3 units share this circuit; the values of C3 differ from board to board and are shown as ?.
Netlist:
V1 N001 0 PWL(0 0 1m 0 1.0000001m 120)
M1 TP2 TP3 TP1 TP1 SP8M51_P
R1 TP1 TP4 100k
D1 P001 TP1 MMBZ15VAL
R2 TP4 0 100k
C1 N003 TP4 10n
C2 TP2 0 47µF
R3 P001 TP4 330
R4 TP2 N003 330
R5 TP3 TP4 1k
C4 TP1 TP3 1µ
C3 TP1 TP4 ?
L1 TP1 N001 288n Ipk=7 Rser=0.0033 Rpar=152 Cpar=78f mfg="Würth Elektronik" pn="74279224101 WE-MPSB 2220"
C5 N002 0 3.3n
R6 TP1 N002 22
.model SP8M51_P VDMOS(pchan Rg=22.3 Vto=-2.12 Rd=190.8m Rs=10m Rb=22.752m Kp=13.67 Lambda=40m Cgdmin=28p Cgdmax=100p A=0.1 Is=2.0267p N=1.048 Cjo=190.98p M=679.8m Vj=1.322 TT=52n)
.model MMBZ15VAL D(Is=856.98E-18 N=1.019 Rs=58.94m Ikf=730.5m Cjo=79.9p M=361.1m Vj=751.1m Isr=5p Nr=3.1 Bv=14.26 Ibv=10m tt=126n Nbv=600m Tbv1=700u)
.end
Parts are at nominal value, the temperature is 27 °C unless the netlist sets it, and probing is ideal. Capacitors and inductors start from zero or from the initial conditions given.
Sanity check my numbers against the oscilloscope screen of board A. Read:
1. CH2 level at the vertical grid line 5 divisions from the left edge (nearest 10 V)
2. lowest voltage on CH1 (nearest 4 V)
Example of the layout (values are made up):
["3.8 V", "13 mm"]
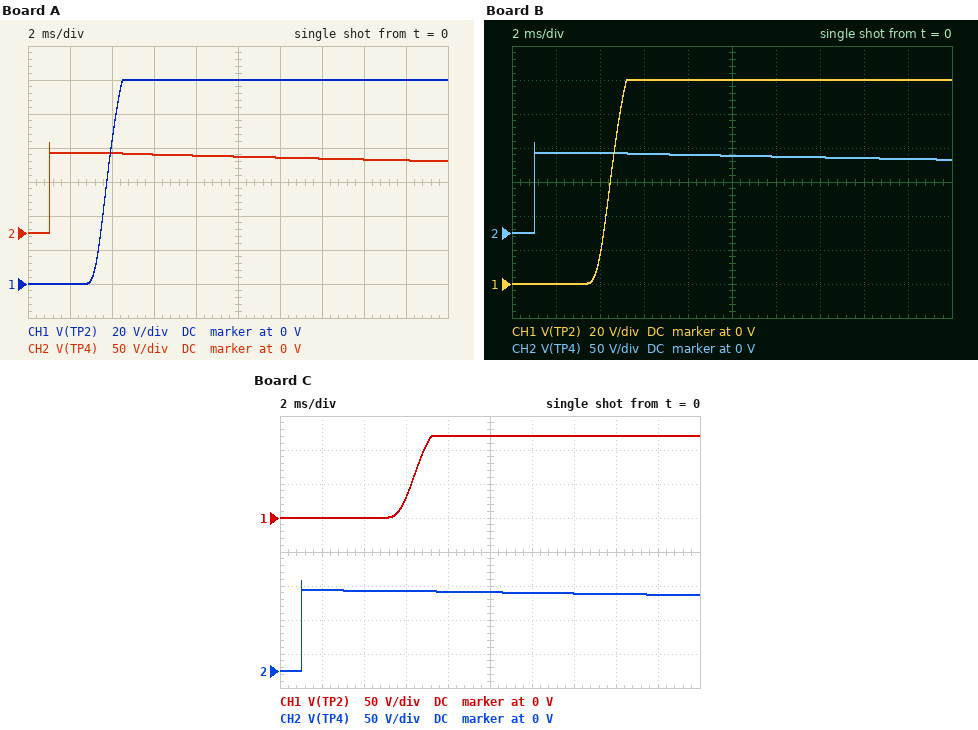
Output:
["110 V", "0 V"]
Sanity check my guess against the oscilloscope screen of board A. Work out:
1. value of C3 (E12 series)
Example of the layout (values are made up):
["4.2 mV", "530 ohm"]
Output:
["390 nF"]
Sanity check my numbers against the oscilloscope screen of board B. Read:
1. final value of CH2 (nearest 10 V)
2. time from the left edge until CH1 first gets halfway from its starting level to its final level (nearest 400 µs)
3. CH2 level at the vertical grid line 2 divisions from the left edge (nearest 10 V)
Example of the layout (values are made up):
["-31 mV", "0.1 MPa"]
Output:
["110 V", "4.4 ms", "120 V"]
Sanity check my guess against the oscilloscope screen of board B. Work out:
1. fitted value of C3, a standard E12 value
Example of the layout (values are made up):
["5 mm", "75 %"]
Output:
["680 nF"]
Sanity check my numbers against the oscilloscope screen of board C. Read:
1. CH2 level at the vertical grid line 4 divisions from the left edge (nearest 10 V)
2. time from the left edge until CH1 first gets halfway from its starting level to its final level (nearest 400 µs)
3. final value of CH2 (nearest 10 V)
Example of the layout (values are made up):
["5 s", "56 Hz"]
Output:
["120 V", "6.4 ms", "110 V"]
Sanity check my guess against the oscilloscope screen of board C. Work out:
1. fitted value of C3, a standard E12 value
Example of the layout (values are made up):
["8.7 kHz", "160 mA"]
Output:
["1.5 µF"]
